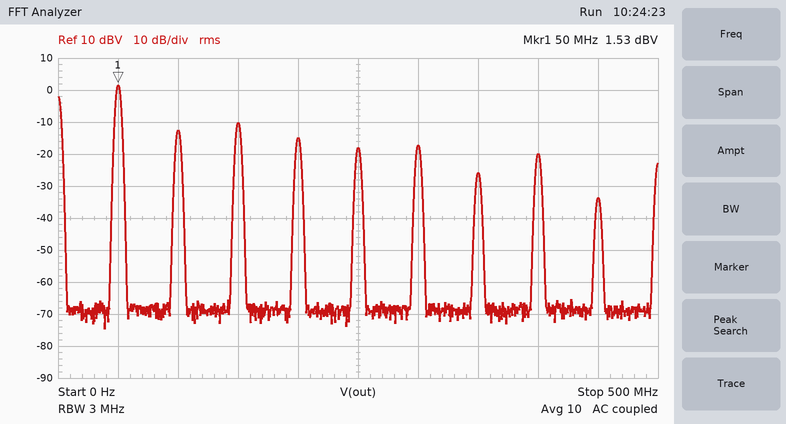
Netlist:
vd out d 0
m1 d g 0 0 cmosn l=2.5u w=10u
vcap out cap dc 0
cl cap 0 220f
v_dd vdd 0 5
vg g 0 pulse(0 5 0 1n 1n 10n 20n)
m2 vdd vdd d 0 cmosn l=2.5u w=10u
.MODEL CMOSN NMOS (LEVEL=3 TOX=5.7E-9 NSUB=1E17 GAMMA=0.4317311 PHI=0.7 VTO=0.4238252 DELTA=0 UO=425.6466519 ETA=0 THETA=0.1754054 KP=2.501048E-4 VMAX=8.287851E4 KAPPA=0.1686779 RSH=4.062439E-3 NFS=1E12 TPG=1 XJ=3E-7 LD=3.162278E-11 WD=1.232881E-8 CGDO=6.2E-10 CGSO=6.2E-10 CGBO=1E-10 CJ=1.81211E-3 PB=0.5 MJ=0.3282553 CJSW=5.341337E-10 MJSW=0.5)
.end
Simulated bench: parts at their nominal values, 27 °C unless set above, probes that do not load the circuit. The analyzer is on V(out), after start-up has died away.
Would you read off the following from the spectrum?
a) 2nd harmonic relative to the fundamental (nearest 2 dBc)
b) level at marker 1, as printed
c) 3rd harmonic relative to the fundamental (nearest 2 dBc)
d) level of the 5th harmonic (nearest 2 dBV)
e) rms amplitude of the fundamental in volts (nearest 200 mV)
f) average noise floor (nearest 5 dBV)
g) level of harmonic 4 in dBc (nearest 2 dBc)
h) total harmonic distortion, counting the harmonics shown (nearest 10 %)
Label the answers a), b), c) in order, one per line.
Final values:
a) -14 dBc
b) 1.53 dBV
c) -12 dBc
d) -18 dBV
e) 1.2 V
f) -70 dBV
g) -16 dBc
h) 40 %
